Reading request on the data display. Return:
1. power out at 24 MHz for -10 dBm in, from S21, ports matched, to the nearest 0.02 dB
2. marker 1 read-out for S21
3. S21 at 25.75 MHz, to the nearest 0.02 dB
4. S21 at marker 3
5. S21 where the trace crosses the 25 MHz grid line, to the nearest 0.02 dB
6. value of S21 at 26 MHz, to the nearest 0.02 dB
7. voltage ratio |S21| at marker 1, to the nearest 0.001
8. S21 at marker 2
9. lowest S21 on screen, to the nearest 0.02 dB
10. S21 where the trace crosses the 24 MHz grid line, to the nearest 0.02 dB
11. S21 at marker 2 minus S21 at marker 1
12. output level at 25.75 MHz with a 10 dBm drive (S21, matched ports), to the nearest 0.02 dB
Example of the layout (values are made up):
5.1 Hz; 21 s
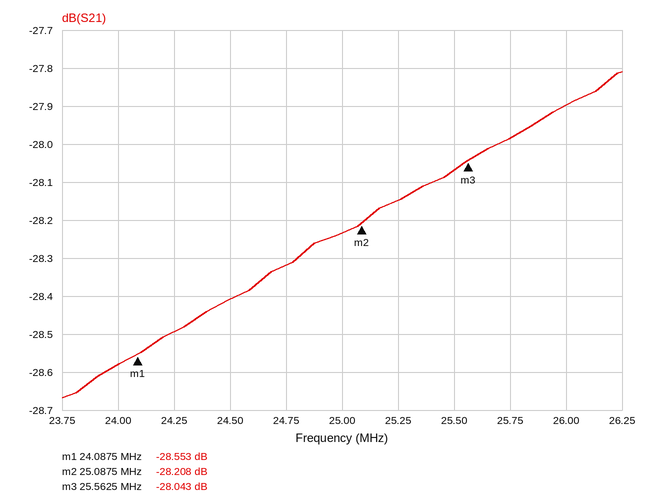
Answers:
-38.58 dBm; -28.553 dB; -27.98 dB; -28.043 dB; -28.24 dB; -27.90 dB; 0.037; -28.208 dB; -28.66 dB; -28.58 dB; 0.345 dB; -17.98 dBm
